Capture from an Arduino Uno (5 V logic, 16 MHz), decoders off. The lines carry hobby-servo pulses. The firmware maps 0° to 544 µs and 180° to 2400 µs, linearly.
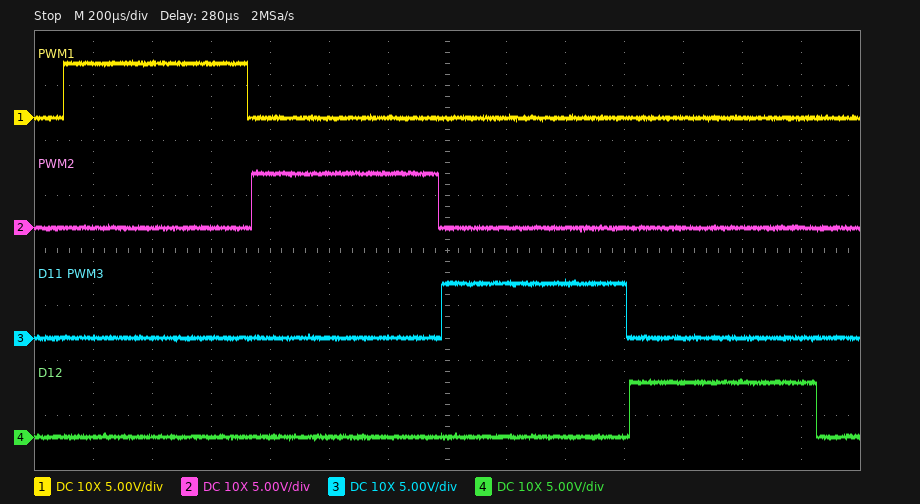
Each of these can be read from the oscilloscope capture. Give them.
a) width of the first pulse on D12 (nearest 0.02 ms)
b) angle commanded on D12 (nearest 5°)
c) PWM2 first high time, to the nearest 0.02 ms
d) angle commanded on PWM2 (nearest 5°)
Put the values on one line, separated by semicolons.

0.64 ms; 10°; 0.64 ms; 10°
